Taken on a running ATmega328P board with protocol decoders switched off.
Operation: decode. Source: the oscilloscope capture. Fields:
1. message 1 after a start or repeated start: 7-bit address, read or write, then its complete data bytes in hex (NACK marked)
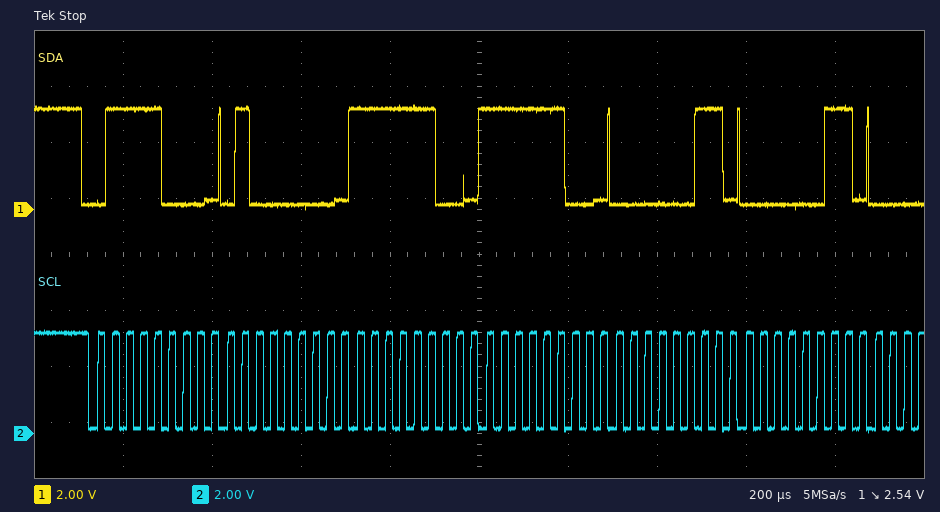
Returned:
0x3C write: 40 FC FC 03 03
